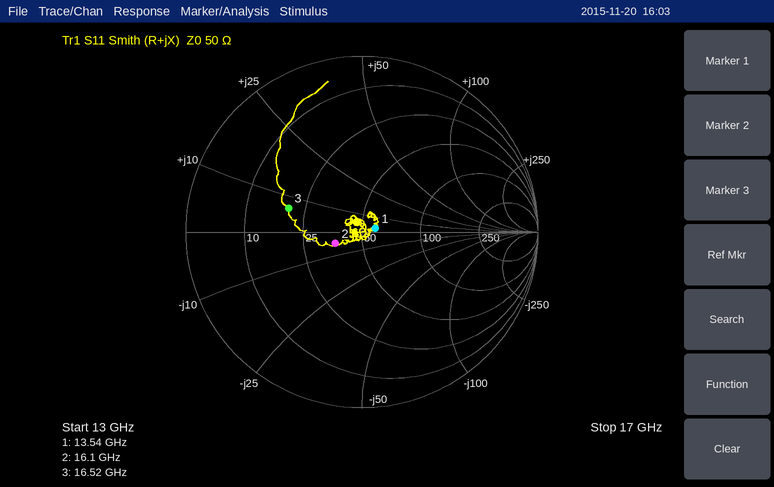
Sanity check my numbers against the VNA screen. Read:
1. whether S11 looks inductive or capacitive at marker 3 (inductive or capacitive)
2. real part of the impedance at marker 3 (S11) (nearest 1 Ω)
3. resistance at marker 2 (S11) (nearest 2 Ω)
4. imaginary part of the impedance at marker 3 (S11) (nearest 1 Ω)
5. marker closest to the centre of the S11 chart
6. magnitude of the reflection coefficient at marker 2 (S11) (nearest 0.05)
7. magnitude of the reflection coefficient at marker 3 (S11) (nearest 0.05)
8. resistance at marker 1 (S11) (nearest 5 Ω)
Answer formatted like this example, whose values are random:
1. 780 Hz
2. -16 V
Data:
1. inductive
2. 20 Ω
3. 36 Ω
4. +7 Ω
5. marker 1
6. 0.15
7. 0.45
8. 60 Ω
